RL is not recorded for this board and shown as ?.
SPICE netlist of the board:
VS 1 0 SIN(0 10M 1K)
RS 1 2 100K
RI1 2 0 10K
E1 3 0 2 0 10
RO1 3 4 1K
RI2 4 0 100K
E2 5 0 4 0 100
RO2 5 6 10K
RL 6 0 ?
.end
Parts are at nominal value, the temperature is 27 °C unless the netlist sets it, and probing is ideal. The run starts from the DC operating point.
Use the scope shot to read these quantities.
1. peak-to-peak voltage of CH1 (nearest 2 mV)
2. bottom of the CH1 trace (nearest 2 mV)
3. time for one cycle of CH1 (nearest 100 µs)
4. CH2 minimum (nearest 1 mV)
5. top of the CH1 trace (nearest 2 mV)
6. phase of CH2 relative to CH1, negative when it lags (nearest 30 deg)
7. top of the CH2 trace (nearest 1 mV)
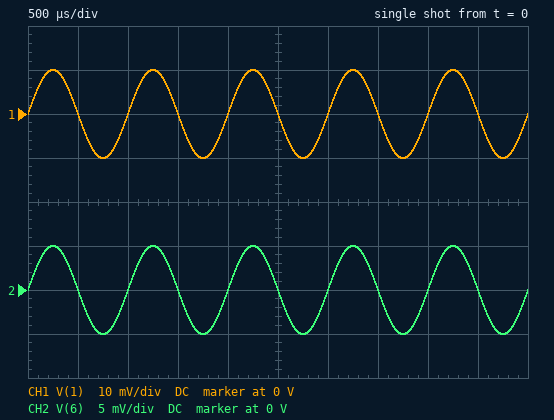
20 mV
-10 mV
1.0 ms
-5 mV
10 mV
0 deg
5 mV
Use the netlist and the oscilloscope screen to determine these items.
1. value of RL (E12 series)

56 Ω
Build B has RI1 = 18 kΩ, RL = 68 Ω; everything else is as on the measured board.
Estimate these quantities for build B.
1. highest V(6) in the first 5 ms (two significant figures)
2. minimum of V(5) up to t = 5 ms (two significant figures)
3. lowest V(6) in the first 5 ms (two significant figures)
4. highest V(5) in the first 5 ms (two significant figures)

10 mV
-1.5 V
-10 mV
1.5 V
